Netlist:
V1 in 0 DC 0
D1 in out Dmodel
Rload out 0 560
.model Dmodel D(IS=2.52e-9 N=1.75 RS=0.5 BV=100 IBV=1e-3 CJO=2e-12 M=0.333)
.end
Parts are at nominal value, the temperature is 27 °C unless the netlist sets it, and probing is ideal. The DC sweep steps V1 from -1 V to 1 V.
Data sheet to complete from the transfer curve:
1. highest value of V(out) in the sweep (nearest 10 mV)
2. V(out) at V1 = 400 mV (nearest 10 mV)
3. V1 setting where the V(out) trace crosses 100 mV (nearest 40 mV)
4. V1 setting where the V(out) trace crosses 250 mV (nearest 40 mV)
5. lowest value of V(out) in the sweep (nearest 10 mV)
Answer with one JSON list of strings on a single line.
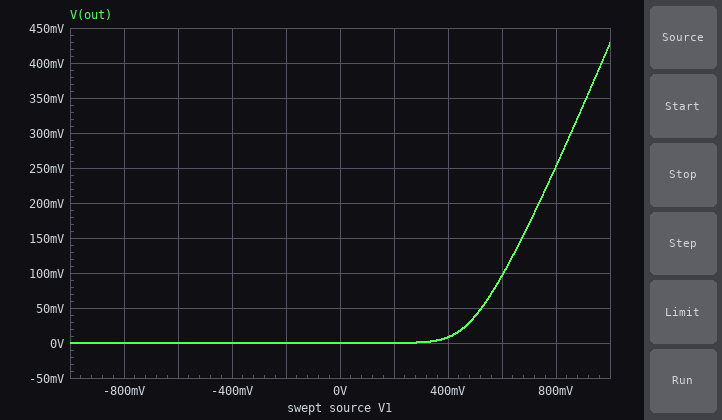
["430 mV", "10 mV", "600 mV", "800 mV", "0 V"]
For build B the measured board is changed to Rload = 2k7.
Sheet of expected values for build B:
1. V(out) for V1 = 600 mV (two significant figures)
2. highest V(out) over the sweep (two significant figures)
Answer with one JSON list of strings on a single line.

["150 mV", "490 mV"]
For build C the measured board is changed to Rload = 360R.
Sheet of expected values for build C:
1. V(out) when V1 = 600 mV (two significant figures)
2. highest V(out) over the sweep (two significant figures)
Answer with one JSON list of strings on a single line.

["83 mV", "410 mV"]
